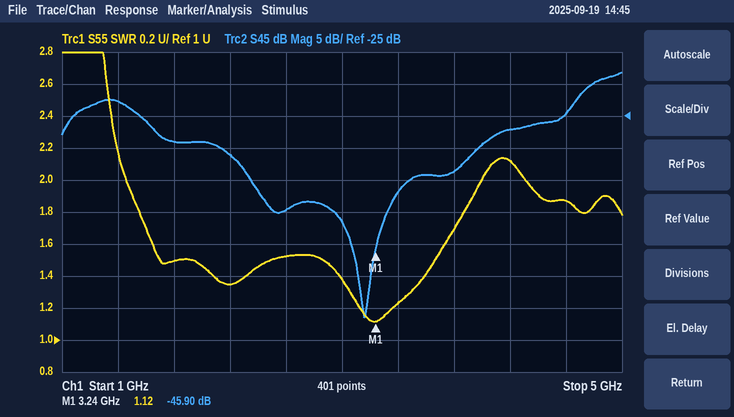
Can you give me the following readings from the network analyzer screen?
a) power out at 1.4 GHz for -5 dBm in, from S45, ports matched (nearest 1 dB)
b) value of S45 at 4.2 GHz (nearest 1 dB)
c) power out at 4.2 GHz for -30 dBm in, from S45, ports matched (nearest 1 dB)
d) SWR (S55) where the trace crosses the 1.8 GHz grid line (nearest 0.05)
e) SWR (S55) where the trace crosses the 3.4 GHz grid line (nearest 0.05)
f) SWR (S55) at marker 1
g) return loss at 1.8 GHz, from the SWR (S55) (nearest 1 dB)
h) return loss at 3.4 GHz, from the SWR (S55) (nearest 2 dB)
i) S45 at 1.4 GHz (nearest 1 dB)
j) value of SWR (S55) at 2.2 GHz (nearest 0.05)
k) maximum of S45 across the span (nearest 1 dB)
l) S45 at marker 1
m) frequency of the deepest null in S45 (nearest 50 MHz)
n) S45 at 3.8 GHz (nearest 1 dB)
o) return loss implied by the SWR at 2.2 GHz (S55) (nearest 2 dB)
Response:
-28 dBm
-27 dB
-57 dBm
1.50
1.25
1.12
14 dB
20 dB
-23 dB
1.35
-18 dB
-45.90 dB
3.15 GHz
-34 dB
16 dB
